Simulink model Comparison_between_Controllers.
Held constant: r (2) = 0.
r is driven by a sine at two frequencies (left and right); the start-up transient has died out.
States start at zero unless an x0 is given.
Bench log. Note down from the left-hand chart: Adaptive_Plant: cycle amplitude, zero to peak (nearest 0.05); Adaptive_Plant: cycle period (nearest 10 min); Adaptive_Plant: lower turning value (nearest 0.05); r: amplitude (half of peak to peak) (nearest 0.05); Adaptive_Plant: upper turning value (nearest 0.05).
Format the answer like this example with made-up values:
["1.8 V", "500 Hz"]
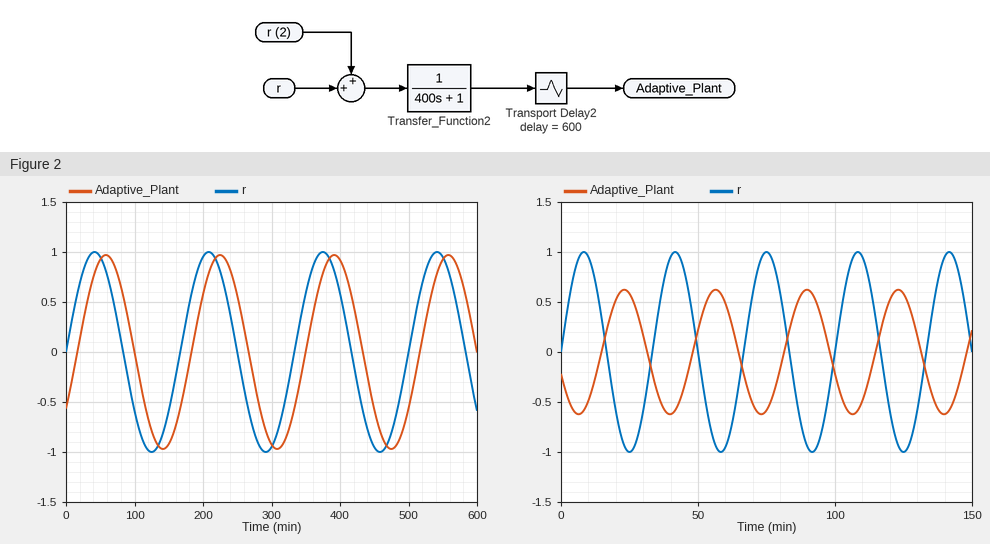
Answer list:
["0.95", "170 min", "-0.95", "1.00", "0.95"]
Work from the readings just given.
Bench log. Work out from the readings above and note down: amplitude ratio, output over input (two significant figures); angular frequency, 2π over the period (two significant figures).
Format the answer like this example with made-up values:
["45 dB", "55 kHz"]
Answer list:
["0.95", "0.037 rad/min"]
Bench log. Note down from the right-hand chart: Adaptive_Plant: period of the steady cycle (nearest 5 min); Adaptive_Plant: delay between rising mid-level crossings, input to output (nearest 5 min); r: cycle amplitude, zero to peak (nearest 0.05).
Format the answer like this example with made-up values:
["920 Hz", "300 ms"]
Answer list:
["35 min", "15 min", "1.00"]
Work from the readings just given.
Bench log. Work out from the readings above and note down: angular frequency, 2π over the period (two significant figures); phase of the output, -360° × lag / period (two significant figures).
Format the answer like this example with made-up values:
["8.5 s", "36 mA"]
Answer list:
["0.18 rad/min", "-150°"]
